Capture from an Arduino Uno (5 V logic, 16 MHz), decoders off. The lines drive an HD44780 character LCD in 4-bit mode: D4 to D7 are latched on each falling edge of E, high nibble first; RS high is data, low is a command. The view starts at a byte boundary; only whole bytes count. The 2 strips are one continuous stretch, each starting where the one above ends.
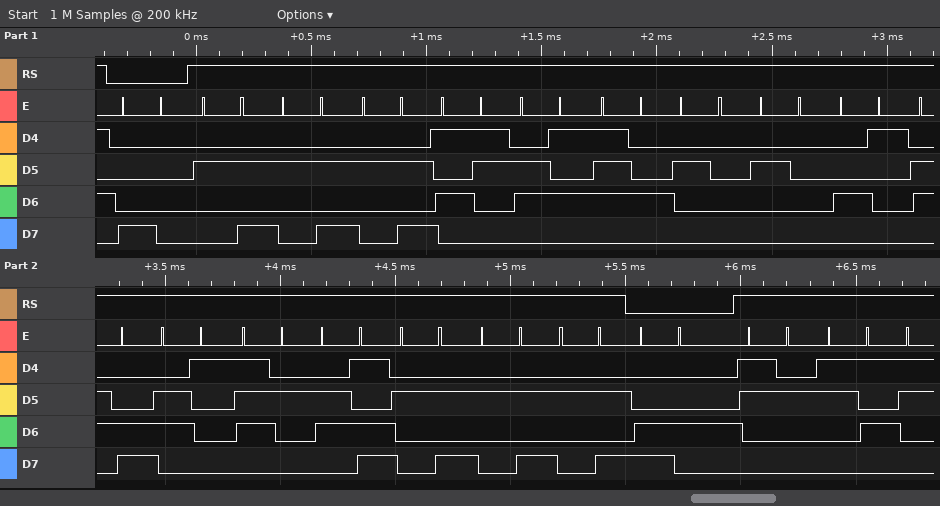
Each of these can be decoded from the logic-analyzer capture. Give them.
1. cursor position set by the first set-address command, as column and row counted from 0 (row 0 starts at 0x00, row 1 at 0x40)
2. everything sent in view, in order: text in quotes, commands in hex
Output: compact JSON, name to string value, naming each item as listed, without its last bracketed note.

{"cursor position set by the first set-address command, as column and row counted from 0": "column 0, row 0", "everything sent in view, in order: text in quotes, commands in hex": "0x80 \"***Set  Alarm***\" 0xC4 \"25\""}
